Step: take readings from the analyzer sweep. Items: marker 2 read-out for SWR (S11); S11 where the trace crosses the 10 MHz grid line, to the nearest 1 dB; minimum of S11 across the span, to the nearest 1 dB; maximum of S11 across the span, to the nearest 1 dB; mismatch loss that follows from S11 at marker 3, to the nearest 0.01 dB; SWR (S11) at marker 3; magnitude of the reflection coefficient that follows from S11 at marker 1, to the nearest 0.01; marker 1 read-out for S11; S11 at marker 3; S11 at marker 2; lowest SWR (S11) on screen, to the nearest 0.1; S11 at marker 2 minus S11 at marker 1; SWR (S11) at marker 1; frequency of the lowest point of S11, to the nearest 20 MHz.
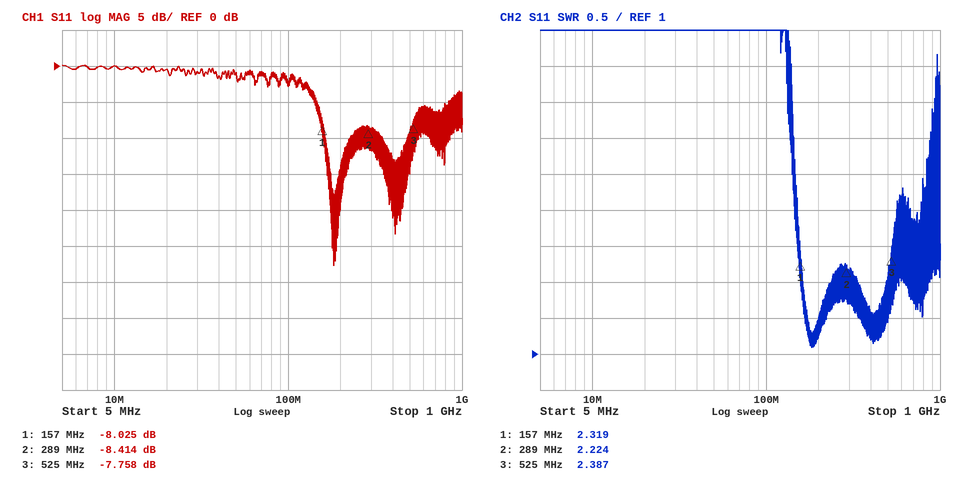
2.224
0 dB
-28 dB
0 dB
0.80 dB
2.387
0.40
-8.025 dB
-7.758 dB
-8.414 dB
1.1
-0.389 dB
2.319
180 MHz
